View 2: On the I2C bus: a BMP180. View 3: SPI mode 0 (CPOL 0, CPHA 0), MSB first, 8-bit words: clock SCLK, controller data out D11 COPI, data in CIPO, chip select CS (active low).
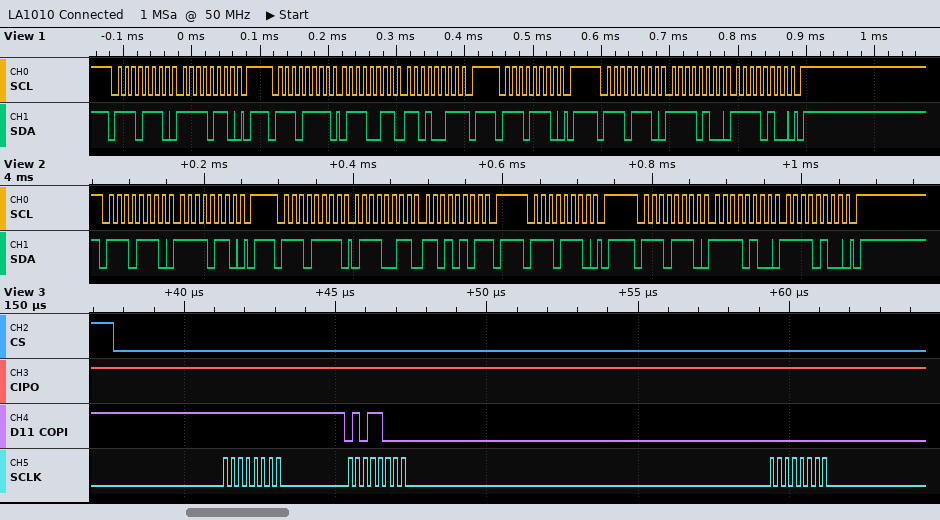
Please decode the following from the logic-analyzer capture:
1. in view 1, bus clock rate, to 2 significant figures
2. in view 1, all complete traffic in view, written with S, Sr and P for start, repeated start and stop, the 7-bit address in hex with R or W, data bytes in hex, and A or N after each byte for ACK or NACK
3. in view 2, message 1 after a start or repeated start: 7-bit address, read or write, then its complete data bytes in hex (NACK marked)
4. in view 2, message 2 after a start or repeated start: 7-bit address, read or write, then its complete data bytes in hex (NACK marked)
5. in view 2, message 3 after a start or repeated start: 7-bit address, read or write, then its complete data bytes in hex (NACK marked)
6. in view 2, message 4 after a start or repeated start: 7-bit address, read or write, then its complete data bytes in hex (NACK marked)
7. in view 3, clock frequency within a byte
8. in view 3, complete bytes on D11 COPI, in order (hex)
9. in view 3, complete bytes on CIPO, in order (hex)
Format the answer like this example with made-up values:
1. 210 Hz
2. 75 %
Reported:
1. 100 kHz
2. S 77W A F6 A P S 77R A 73 A D3 N P S 77W A P S 77W A F4 A F4 A P
3. 0x77 write: F6
4. 0x77 read: 73 D5 NACK
5. 0x77 write
6. 0x77 write: F4 F4
7. 4 MHz
8. FF 58 00
9. FF FF FF
